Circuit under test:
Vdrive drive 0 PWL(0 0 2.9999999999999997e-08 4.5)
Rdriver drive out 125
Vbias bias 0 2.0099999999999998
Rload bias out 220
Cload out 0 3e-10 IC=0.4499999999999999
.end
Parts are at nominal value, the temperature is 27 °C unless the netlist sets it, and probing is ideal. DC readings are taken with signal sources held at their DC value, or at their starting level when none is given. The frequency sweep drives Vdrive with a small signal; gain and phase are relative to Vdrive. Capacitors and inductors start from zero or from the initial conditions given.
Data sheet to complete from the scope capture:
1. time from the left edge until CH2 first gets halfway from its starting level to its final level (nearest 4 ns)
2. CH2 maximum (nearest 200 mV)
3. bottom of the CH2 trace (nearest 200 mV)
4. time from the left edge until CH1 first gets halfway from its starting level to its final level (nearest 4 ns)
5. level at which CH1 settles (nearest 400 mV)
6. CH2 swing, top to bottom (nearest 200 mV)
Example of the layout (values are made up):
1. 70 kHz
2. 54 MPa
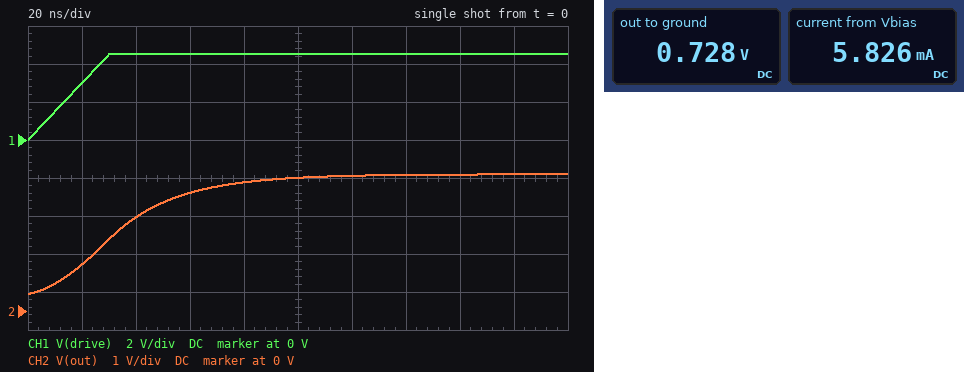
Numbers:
1. 32 ns
2. 3.6 V
3. 400 mV
4. 16 ns
5. 4.4 V
6. 3.2 V
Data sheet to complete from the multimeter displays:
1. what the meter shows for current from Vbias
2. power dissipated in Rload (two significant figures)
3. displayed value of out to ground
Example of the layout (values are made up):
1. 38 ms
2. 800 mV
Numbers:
1. 5.826 mA
2. 7.5 mW
3. 0.728 V
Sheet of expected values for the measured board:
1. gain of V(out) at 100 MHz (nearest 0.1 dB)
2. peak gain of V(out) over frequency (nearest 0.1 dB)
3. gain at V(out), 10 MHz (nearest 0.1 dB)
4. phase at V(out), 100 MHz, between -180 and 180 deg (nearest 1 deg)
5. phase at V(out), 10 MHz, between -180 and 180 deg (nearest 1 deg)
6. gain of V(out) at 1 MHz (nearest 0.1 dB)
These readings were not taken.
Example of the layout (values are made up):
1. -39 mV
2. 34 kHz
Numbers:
1. -27.5 dB
2. -3.9 dB
3. -9.0 dB
4. -86 deg
5. -56 deg
6. -4.0 dB
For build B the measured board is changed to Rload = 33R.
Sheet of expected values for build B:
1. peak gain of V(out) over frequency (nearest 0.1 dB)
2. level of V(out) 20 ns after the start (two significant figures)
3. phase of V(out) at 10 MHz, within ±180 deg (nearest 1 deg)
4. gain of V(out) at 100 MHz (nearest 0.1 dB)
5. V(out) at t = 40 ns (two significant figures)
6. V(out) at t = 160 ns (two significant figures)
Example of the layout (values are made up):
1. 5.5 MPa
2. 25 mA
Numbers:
1. -13.6 dB
2. 1.9 V
3. -26 deg
4. -27.6 dB
5. 2.5 V
6. 2.5 V
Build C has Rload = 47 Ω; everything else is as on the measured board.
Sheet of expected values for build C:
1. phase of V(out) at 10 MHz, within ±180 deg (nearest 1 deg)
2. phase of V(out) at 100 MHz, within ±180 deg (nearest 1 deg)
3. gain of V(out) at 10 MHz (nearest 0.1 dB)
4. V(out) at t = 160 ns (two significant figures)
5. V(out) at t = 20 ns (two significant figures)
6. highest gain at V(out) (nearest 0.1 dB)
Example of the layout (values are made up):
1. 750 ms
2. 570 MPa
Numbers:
1. -33 deg
2. -81 deg
3. -12.8 dB
4. 2.7 V
5. 1.8 V
6. -11.3 dB
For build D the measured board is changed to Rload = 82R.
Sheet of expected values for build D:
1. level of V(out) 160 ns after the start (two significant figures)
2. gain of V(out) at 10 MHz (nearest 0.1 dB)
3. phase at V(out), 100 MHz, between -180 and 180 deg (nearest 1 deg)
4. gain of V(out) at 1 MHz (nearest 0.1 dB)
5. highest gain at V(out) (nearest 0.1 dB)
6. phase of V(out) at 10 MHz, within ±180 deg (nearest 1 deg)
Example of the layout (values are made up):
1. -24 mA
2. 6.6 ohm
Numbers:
1. 3.0 V
2. -10.8 dB
3. -84 deg
4. -8.1 dB
5. -8.0 dB
6. -43 deg
